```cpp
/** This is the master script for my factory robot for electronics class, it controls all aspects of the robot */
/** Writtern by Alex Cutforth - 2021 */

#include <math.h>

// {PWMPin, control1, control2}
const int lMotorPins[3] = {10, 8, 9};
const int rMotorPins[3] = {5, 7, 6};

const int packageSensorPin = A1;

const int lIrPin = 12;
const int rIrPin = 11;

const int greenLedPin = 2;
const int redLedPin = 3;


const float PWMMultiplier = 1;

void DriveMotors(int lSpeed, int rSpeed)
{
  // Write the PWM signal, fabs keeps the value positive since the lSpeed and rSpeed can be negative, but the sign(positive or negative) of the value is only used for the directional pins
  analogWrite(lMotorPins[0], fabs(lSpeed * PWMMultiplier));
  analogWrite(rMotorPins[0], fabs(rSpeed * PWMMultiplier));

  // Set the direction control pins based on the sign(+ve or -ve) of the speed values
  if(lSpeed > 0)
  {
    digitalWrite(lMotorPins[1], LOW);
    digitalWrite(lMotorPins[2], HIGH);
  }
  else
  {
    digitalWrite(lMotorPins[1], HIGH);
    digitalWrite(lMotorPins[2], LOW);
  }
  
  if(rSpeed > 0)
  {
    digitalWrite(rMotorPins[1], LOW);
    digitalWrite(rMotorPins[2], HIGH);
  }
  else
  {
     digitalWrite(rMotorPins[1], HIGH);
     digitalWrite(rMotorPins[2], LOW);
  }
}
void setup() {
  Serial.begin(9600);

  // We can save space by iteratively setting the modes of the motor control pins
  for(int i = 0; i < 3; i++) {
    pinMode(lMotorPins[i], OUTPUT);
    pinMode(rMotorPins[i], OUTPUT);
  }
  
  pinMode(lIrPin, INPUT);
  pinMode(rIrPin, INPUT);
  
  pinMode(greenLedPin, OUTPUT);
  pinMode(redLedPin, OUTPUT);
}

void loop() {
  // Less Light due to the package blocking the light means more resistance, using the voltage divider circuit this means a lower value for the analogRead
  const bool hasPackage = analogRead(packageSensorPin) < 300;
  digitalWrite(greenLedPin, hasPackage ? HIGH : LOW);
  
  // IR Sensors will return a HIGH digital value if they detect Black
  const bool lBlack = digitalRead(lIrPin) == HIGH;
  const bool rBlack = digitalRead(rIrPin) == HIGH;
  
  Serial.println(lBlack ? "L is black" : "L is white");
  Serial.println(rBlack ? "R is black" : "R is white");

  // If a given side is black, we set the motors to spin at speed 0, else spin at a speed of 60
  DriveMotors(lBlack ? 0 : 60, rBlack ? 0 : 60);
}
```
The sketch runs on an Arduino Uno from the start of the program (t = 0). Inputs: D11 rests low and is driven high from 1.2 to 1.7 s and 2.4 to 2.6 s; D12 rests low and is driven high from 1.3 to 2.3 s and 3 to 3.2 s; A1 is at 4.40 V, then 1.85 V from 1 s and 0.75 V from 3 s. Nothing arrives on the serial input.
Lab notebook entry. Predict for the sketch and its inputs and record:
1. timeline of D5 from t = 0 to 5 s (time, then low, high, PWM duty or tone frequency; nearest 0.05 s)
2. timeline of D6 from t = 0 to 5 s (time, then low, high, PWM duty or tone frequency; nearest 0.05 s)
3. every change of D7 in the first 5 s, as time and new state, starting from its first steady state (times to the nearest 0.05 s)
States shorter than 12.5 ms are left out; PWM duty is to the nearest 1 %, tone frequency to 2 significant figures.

0 s PWM 24 %; 1.25 s low; 1.75 s PWM 24 %; 2.45 s low; 2.65 s PWM 24 %
0 s high; 1.25 s low; 1.75 s high; 2.45 s low; 2.65 s high
0 s low; 1.25 s high; 1.75 s low; 2.45 s high; 2.65 s low
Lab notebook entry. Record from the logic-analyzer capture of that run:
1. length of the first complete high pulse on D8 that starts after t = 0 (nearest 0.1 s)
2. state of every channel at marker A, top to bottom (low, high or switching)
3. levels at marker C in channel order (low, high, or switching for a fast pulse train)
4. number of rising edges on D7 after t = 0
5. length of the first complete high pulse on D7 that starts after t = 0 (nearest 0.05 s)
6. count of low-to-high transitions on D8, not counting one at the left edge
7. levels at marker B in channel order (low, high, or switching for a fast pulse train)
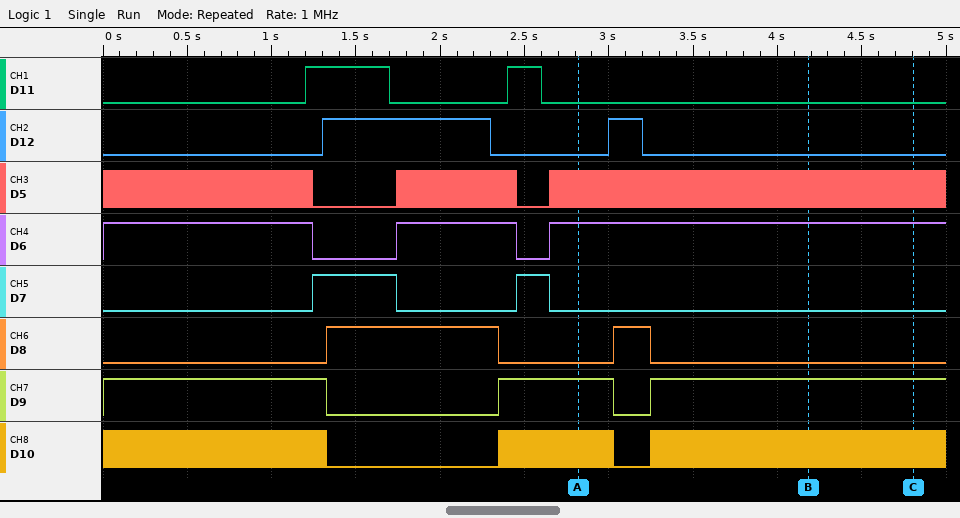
1.0 s
D11 low, D12 low, D5 switching, D6 high, D7 low, D8 low, D9 high, D10 switching
D11 low, D12 low, D5 switching, D6 high, D7 low, D8 low, D9 high, D10 switching
2
0.50 s
2
D11 low, D12 low, D5 switching, D6 high, D7 low, D8 low, D9 high, D10 switching
